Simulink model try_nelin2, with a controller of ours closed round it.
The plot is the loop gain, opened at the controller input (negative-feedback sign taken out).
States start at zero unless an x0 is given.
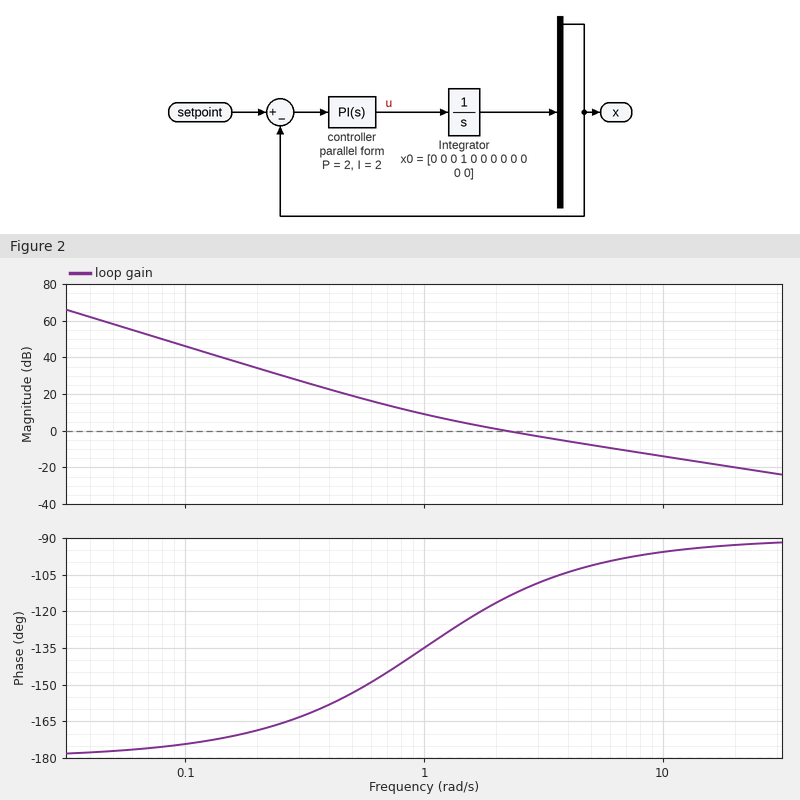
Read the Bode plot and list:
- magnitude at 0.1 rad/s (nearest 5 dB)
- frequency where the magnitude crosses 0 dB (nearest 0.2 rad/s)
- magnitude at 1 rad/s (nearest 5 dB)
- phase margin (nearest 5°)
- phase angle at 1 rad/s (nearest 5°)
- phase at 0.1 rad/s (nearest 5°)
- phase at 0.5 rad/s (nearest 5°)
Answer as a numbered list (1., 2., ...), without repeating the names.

1. 45 dB
2. 2.2 rad/s
3. 10 dB
4. 65°
5. -135°
6. -175°
7. -155°
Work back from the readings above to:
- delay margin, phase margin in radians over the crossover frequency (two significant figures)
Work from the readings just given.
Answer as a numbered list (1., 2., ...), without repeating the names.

1. 0.52 s
